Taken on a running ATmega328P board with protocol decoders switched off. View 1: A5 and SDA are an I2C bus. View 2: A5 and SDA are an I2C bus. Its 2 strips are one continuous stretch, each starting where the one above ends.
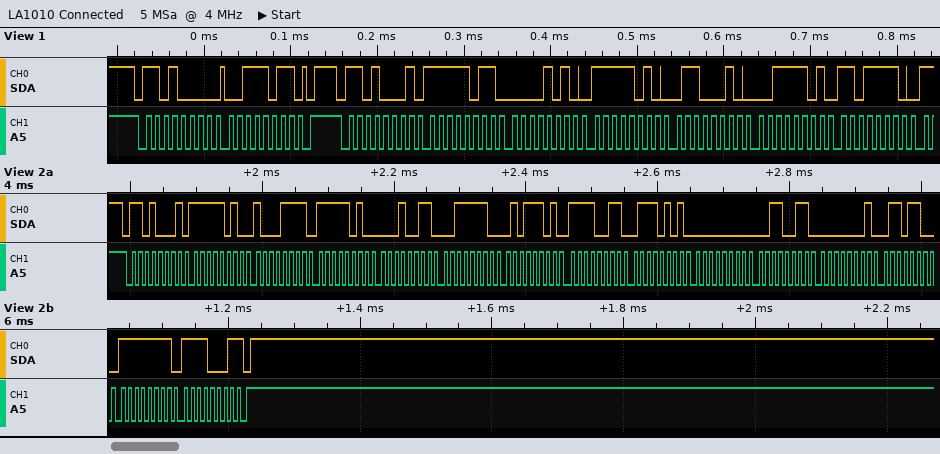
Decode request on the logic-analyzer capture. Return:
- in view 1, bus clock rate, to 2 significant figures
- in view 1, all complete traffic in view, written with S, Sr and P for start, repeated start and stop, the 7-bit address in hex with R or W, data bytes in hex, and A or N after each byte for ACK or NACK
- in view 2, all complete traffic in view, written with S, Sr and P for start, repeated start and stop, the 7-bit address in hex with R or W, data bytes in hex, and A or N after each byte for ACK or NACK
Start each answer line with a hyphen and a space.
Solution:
- 100 kHz
- S 68W A 3B A P S 68R A FB A 0A A FA A 62 A 3D A DE A
- S 68R A FA A 8F A FA A 13 A 3E A 5D A F3 A 75 A 00 A 33 A 01 A 6C A FF A F1 N P
